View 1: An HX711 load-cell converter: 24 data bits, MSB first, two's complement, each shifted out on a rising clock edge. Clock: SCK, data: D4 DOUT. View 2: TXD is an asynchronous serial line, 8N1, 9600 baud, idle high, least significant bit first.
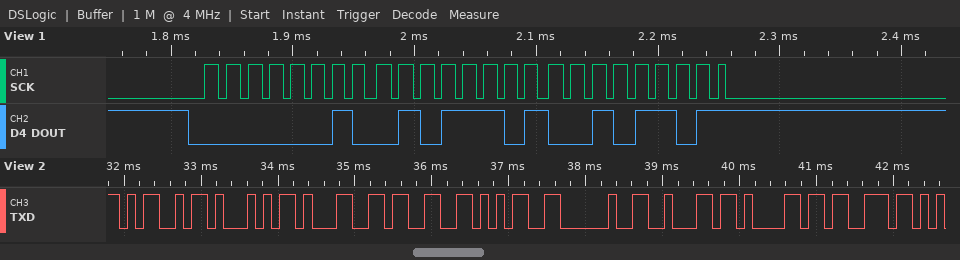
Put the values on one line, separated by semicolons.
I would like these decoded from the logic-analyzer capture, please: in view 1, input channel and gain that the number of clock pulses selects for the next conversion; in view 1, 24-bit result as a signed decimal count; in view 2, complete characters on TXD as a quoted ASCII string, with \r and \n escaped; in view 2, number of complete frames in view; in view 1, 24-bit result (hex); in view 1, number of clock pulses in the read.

channel A, gain 128; 154925; "MQ135 bas"; 9; 0x025D2D; 25
